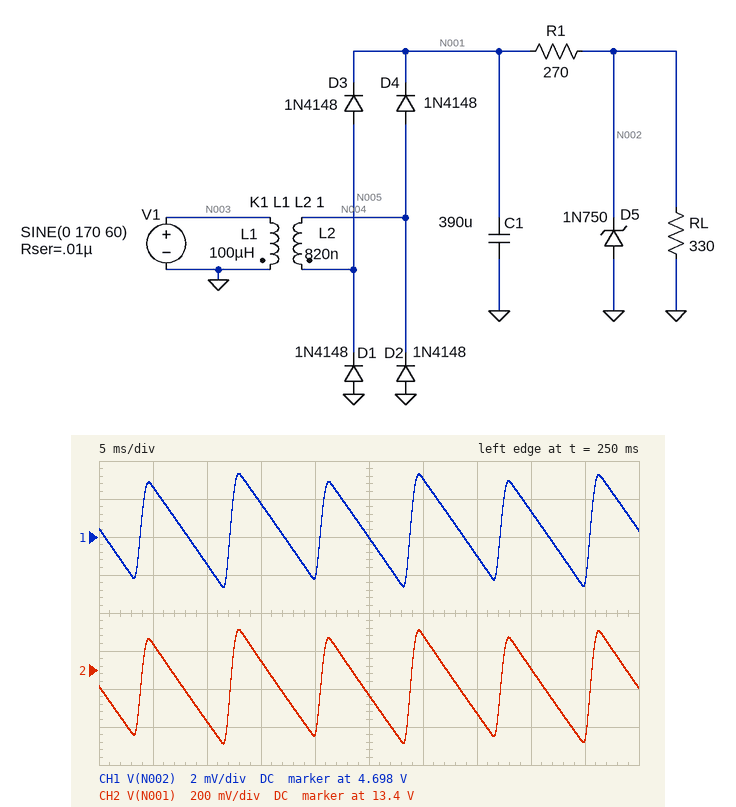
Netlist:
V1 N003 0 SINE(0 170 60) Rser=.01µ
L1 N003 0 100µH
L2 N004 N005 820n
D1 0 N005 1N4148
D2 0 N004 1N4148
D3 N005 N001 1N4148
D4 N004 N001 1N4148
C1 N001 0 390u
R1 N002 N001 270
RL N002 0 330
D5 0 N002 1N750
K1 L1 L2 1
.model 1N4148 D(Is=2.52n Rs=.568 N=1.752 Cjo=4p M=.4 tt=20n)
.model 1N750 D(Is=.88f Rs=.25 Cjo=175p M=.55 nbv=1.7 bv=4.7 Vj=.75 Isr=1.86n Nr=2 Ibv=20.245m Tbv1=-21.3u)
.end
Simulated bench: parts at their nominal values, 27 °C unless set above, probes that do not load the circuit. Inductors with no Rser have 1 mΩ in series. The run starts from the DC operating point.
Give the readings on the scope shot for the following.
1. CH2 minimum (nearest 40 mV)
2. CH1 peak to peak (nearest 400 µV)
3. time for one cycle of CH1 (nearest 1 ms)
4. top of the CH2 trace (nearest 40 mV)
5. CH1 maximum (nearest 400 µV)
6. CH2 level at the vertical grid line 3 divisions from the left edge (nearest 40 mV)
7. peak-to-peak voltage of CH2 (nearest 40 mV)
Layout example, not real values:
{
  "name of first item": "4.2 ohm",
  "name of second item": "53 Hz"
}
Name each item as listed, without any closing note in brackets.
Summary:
{
  "CH2 minimum": "13.00 V",
  "CH1 peak to peak": "6.0 mV",
  "time for one cycle of CH1": "8 ms",
  "top of the CH2 trace": "13.60 V",
  "CH1 maximum": "4.7012 V",
  "CH2 level at the vertical grid line 3 divisions from the left edge": "13.44 V",
  "peak-to-peak voltage of CH2": "600 mV"
}
